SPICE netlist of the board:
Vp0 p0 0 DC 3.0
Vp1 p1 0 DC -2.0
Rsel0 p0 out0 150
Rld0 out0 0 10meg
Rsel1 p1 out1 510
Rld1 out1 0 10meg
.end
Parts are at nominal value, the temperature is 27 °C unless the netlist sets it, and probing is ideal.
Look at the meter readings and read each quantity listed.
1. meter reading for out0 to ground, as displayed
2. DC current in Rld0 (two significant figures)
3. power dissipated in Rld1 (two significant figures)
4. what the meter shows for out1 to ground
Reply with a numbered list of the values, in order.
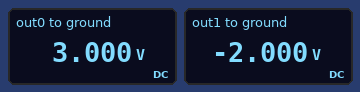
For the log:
1. 3.000 V
2. 300 nA
3. 400 nW
4. -2.000 V
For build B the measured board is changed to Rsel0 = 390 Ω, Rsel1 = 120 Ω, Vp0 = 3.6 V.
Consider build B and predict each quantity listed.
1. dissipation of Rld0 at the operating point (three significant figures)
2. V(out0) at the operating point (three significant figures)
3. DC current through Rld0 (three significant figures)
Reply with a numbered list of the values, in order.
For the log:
1. 1.30 µW
2. 3.60 V
3. 360 nA
